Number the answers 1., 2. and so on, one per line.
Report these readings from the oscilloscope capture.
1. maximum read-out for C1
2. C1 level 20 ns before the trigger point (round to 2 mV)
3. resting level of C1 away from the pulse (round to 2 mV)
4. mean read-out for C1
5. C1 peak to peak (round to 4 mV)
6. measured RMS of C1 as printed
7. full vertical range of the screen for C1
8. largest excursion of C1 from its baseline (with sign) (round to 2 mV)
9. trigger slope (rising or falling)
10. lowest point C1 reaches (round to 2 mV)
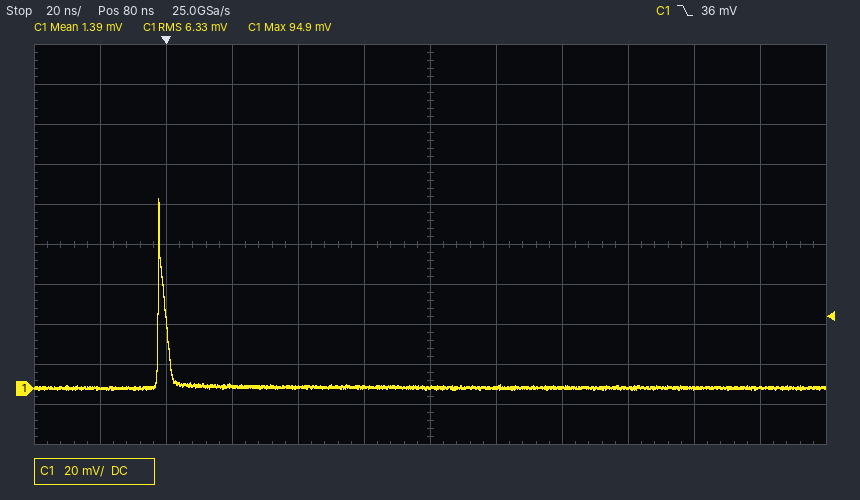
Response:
1. 94.9 mV
2. 0 mV
3. 0 mV
4. 1.39 mV
5. 96 mV
6. 6.33 mV
7. 200 mV
8. +94 mV
9. falling
10. 0 mV
